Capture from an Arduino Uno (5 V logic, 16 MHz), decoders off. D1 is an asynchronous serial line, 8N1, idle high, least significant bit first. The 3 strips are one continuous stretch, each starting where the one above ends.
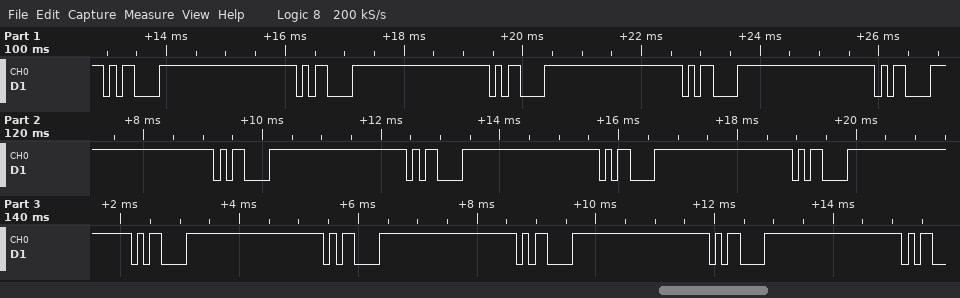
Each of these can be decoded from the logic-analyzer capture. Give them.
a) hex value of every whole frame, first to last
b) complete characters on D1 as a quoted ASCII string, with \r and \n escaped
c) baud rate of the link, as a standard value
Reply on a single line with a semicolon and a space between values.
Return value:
0D 0D 0D 0D 0D 0D 0D 0D 0D 0D 0D 0D 0D; "\r\r\r\r\r\r\r\r\r\r\r\r\r"; 9600 baud
